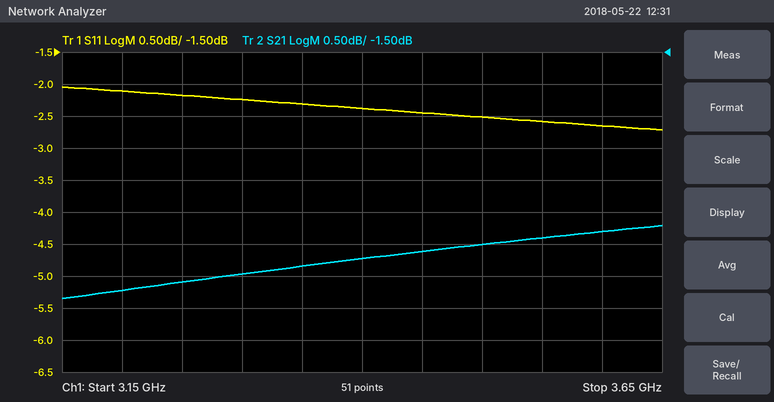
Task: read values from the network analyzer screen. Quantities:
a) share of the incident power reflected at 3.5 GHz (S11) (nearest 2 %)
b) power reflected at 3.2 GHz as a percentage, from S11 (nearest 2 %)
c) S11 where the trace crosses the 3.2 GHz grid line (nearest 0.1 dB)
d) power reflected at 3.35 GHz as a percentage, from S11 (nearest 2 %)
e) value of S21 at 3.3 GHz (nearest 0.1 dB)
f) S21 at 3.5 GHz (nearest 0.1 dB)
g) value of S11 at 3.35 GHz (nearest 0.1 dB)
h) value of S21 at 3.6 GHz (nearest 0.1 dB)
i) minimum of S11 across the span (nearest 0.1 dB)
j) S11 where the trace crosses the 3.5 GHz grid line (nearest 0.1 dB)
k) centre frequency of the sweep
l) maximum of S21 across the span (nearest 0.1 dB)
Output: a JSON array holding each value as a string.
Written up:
["56 %", "62 %", "-2.1 dB", "58 %", "-5.0 dB", "-4.5 dB", "-2.3 dB", "-4.3 dB", "-2.7 dB", "-2.5 dB", "3.4 GHz", "-4.2 dB"]
